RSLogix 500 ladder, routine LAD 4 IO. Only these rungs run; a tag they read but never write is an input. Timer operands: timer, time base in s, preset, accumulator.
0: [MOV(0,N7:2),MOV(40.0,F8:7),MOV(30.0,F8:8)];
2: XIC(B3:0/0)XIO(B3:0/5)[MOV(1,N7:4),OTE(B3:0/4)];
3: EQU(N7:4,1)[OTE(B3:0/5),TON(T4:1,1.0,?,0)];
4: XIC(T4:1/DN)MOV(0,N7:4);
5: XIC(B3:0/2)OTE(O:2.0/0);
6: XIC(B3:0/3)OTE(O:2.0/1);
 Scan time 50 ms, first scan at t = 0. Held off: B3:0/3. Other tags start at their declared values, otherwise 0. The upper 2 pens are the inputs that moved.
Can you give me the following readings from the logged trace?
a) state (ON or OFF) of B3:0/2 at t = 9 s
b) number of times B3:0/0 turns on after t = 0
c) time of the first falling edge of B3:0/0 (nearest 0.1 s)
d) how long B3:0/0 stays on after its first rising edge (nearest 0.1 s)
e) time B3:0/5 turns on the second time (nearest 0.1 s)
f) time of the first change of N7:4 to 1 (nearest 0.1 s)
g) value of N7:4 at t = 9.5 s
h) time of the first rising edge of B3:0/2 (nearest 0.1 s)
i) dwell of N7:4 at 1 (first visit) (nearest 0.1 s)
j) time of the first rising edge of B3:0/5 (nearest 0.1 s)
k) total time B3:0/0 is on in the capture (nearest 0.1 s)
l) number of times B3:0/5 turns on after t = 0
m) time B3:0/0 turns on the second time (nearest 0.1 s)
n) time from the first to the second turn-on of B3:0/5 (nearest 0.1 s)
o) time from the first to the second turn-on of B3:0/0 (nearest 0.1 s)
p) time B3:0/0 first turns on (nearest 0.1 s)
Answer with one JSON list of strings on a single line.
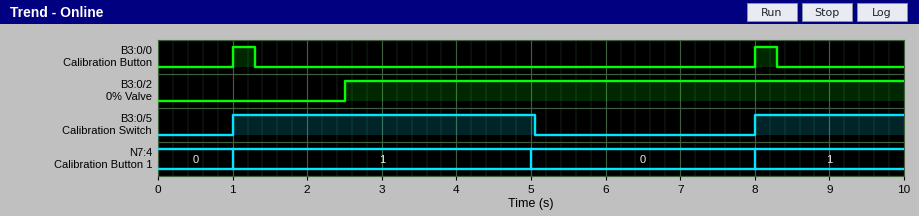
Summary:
["ON", "2", "1.3 s", "0.3 s", "8.0 s", "1.0 s", "1", "2.5 s", "4.0 s", "1.0 s", "0.6 s", "2", "8.0 s", "7.0 s", "7.0 s", "1.0 s"]
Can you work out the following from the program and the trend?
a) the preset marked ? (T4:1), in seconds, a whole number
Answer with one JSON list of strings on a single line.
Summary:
["4 s"]
